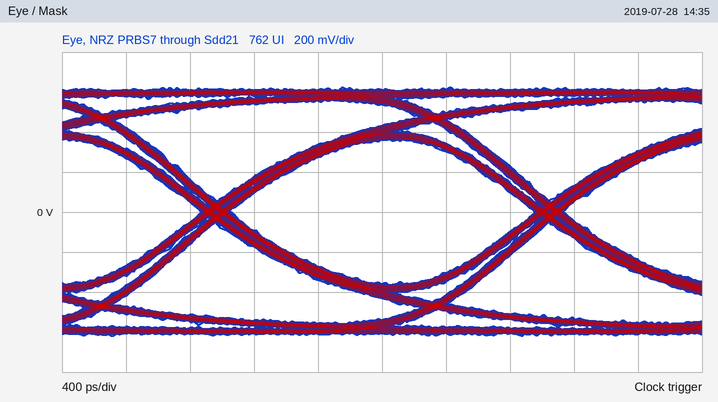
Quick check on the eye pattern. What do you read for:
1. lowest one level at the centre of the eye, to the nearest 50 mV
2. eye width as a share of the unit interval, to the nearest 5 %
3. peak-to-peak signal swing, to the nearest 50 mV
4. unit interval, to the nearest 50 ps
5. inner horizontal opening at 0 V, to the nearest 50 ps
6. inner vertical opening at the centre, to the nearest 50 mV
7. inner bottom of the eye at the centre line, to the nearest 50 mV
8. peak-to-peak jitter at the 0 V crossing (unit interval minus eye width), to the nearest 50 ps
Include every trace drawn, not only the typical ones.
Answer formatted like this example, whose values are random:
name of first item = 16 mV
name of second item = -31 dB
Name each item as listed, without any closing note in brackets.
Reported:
lowest one level at the centre of the eye, to the nearest 50 mV = 350 mV
eye width as a share of the unit interval, to the nearest 5 % = 90 %
peak-to-peak signal swing, to the nearest 50 mV = 1.25 V
unit interval, to the nearest 50 ps = 2.10 ns
inner horizontal opening at 0 V, to the nearest 50 ps = 1.90 ns
inner vertical opening at the centre, to the nearest 50 mV = 700 mV
inner bottom of the eye at the centre line, to the nearest 50 mV = -350 mV
peak-to-peak jitter at the 0 V crossing (unit interval minus eye width), to the nearest 50 ps = 200 ps
